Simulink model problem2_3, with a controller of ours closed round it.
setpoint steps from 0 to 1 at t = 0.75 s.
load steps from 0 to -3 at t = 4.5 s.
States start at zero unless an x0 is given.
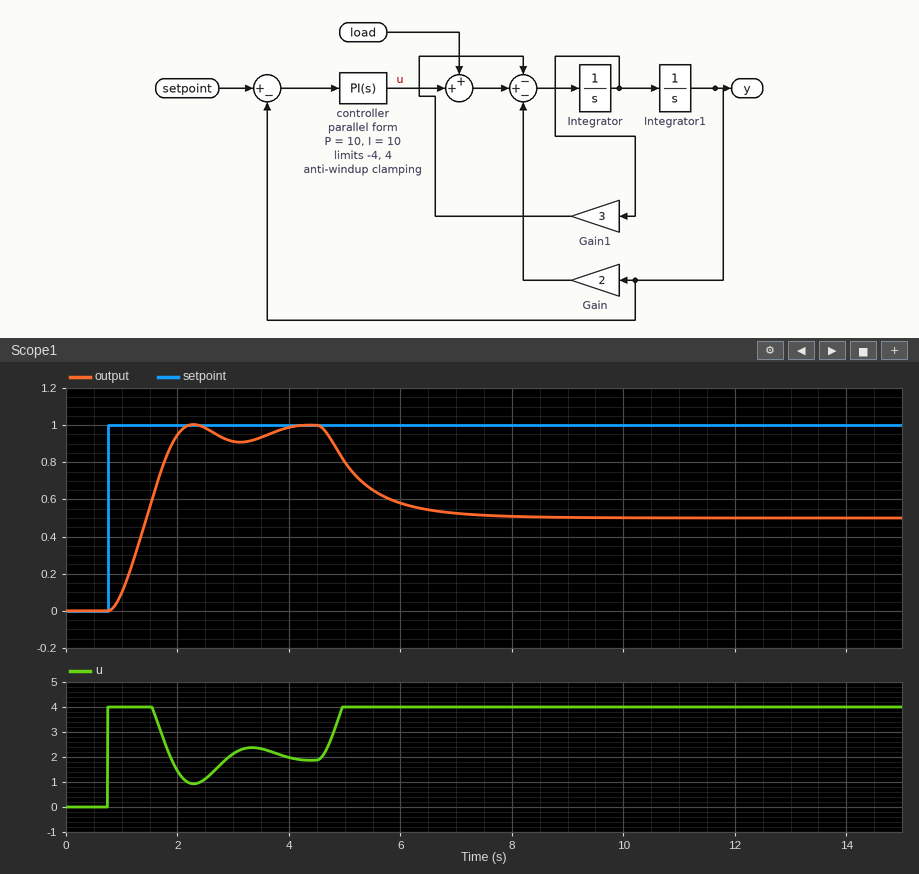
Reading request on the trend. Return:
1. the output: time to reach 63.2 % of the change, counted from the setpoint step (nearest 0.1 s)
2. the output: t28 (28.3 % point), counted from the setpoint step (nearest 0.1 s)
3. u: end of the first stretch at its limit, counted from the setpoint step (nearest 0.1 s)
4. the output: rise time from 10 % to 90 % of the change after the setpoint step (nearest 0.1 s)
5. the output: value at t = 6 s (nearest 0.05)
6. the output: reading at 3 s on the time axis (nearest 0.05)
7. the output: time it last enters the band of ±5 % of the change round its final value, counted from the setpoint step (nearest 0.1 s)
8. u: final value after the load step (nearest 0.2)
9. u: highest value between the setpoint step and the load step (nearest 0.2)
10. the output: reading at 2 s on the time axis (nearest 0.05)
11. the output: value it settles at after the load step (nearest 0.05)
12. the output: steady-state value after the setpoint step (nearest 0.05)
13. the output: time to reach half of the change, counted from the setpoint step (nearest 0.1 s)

0.8 s
0.5 s
0.8 s
0.9 s
0.60
0.90
2.9 s
4.0
4.0
0.95
0.50
1.00
0.7 s
